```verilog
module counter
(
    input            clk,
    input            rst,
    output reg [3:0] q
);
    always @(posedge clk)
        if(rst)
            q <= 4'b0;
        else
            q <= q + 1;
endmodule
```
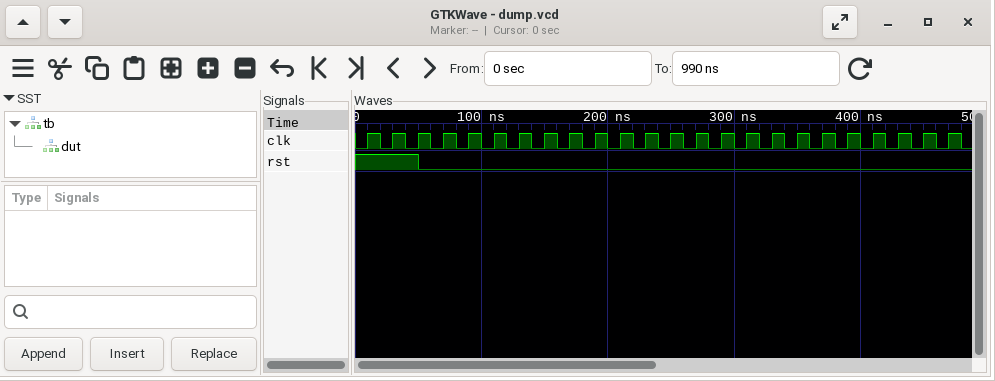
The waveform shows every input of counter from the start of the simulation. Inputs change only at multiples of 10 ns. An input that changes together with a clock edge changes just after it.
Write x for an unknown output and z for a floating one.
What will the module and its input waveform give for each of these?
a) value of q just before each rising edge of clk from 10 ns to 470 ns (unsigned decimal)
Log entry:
x, 0, 0, 0, 1, 2, 3, 4, 5, 6, 7, 8, 9, 10, 11, 12, 13, 14, 15, 0, 1, 2, 3, 4
